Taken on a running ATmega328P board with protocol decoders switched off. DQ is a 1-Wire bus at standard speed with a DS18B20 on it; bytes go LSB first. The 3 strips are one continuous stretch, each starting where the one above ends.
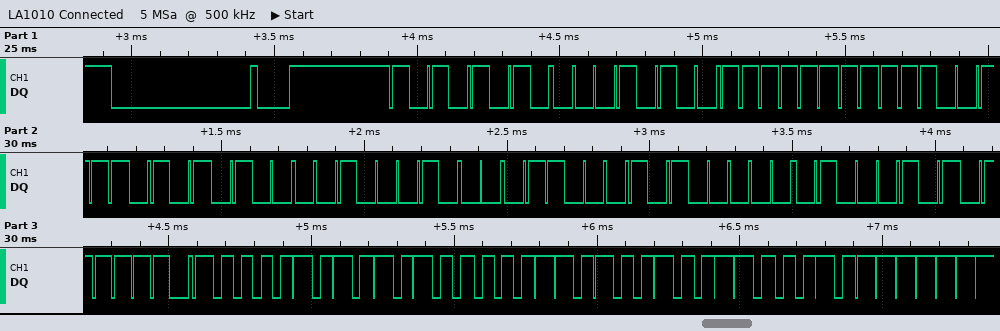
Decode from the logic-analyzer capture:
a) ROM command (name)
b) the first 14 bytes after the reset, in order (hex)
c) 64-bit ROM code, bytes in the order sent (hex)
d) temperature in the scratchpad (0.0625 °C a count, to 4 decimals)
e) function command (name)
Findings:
Match ROM
55 28 FF E7 2A 44 18 05 A2 BE 50 05 4B 46
28 FF E7 2A 44 18 05 A2
85.0000 °C
Read Scratchpad
